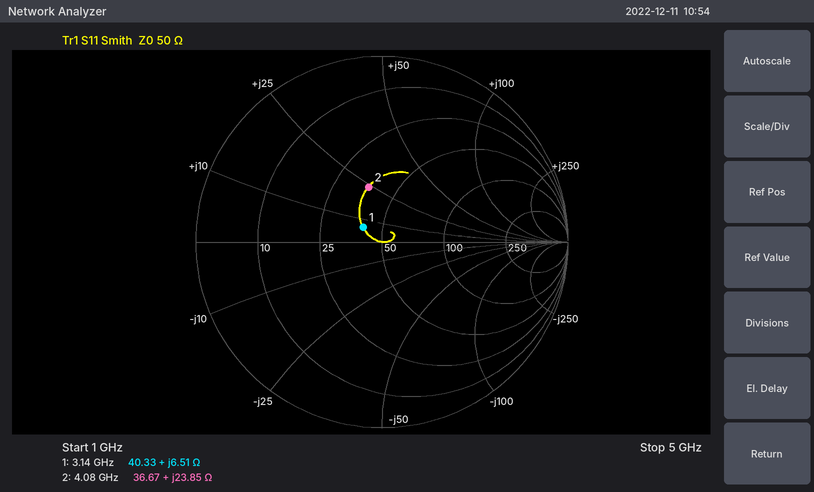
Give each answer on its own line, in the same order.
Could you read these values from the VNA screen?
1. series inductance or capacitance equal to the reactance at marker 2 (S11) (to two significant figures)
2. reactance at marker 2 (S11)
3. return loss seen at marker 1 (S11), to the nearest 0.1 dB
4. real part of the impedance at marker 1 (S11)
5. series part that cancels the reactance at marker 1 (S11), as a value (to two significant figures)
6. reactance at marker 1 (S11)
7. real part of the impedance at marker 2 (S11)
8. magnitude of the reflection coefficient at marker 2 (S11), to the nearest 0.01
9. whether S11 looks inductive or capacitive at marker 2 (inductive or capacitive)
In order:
930 pH
+23.85 Ω
17.8 dB
40.33 Ω
7.8 pF
+6.51 Ω
36.67 Ω
0.30
inductive
